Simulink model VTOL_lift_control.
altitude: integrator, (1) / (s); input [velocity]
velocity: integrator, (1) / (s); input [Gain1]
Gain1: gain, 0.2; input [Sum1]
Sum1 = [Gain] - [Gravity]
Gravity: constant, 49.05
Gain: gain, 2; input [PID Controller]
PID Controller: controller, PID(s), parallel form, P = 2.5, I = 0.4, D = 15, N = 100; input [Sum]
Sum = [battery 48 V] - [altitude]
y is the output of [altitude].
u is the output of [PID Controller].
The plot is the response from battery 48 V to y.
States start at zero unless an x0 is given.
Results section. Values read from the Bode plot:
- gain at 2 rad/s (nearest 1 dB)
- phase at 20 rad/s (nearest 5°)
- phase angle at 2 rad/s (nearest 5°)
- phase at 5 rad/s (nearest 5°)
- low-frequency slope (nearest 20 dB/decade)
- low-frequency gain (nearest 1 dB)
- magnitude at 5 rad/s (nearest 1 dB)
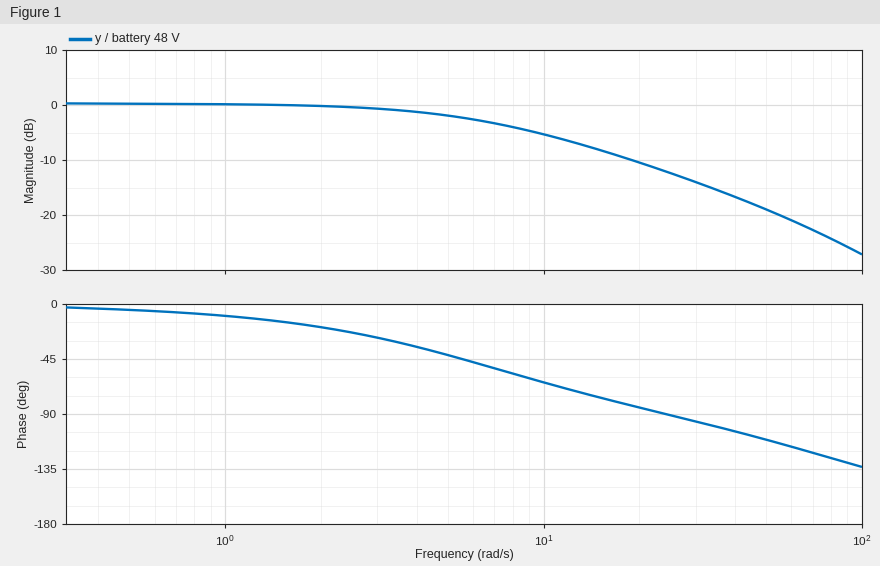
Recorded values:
0 dB
-85°
-20°
-40°
0 dB/decade
0 dB
-2 dB
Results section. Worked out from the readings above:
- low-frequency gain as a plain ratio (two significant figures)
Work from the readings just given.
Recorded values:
1.0
